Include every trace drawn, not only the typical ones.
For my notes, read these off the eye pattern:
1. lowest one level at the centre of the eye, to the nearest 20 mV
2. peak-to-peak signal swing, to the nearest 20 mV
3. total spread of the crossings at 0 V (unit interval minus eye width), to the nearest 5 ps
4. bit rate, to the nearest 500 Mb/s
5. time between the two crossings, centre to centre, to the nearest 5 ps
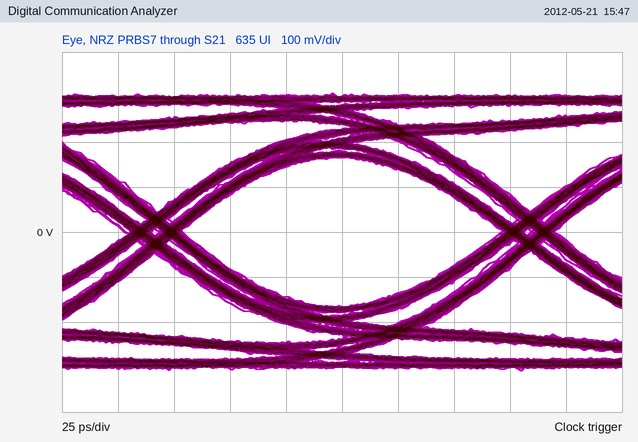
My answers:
160 mV
620 mV
25 ps
6.0 Gb/s
165 ps
